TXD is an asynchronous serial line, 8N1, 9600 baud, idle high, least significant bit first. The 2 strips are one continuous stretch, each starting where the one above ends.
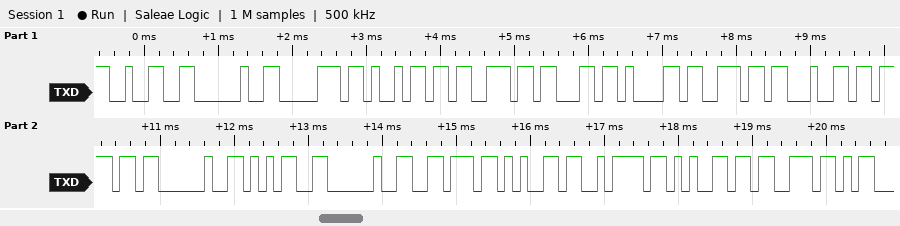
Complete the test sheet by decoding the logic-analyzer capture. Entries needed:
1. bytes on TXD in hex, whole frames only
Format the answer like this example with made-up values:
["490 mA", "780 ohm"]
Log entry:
["0x32 0x20 0x70 0x69 0x73 0x63 0x61 0x6E 0x64 0x6F 0x20 0x35 0x20 0x76 0x65 0x7A 0x65 0x73"]
